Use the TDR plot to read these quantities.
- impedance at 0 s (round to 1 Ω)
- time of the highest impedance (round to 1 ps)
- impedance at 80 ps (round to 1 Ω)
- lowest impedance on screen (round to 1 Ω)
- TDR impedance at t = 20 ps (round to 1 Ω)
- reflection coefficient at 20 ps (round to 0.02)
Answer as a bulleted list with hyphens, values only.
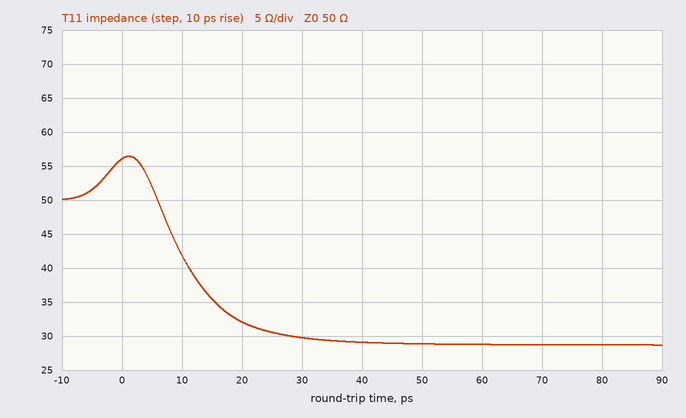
- 56 Ω
- 1 ps
- 29 Ω
- 29 Ω
- 32 Ω
- -0.22
